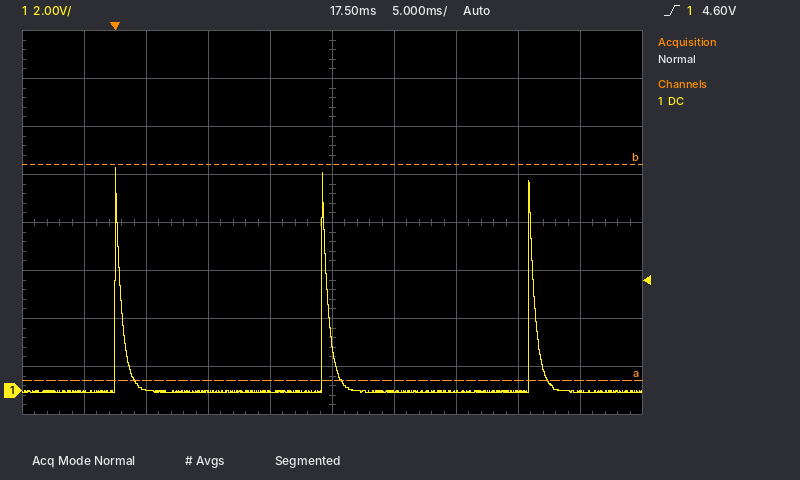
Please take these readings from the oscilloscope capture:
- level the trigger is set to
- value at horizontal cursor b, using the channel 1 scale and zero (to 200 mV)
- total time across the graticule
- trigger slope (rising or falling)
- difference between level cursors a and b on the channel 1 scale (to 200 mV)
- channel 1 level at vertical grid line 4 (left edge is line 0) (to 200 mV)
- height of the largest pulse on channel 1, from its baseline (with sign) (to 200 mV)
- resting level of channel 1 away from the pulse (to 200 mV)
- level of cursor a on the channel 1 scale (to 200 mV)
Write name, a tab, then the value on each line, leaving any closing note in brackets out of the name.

level the trigger is set to	4.60 V
value at horizontal cursor b, using the channel 1 scale and zero	9.4 V
total time across the graticule	50 ms
trigger slope	rising
difference between level cursors a and b on the channel 1 scale	9.0 V
channel 1 level at vertical grid line 4 (left edge is line 0)	0.0 V
height of the largest pulse on channel 1, from its baseline (with sign)	+9.4 V
resting level of channel 1 away from the pulse	0.0 V
level of cursor a on the channel 1 scale	400 mV
